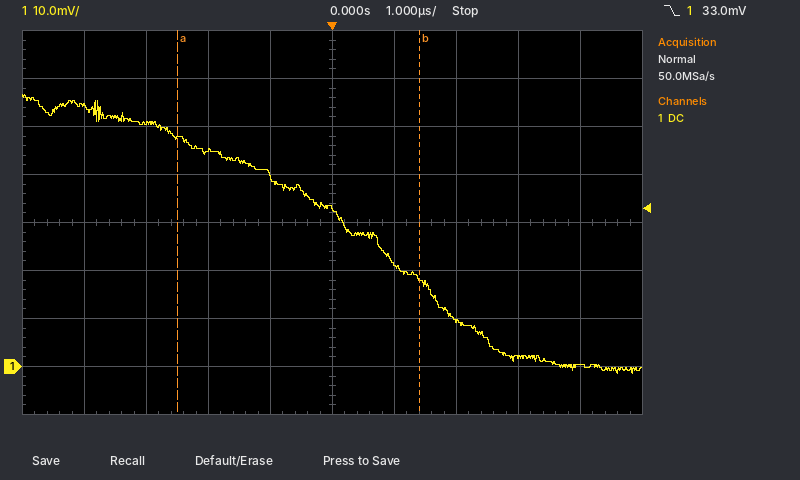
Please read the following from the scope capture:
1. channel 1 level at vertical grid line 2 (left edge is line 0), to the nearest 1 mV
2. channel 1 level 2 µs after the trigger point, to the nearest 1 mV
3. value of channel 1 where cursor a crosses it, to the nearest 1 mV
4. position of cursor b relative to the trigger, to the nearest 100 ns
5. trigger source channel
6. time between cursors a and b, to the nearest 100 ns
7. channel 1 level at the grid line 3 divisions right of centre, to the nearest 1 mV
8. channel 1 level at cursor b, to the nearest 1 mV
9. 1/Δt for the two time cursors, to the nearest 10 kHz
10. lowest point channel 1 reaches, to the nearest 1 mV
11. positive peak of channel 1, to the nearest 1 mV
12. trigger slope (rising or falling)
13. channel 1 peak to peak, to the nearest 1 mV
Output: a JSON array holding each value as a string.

["51 mV", "10 mV", "48 mV", "+1.4 µs", "channel 1", "3.9 µs", "2 mV", "18 mV", "260 kHz", "-1 mV", "57 mV", "falling", "58 mV"]
